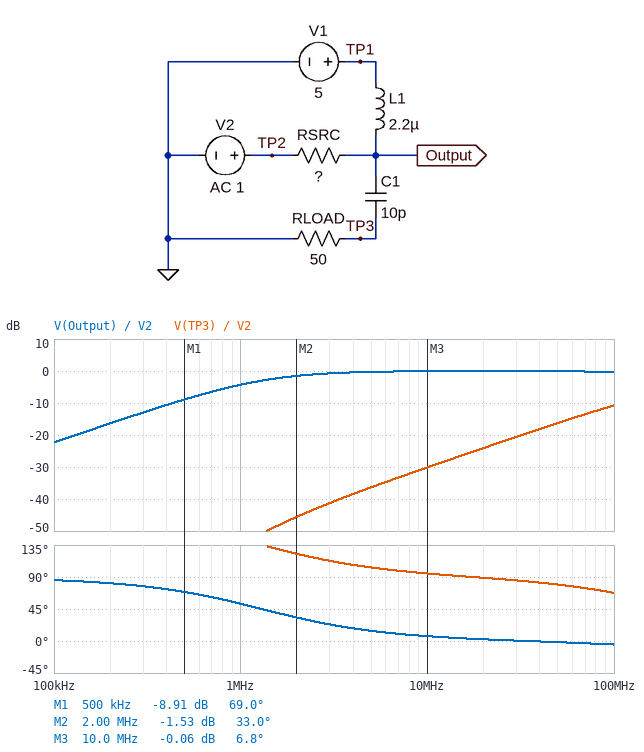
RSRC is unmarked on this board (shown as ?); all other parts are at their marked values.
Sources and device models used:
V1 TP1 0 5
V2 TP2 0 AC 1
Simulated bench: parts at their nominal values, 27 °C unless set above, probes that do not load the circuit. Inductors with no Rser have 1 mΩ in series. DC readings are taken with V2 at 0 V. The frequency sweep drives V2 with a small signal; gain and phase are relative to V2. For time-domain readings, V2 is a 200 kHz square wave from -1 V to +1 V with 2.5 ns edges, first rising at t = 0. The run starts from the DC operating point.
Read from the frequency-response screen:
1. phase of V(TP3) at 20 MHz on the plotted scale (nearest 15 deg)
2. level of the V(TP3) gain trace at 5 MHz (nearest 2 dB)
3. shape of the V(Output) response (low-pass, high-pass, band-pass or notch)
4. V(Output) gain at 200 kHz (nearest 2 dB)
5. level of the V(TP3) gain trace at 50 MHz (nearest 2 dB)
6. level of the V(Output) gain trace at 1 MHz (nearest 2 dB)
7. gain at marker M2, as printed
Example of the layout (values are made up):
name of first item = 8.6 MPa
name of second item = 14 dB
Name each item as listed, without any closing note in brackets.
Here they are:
phase of V(TP3) at 20 MHz on the plotted scale = 90 deg
level of the V(TP3) gain trace at 5 MHz = -36 dB
shape of the V(Output) response = high-pass
V(Output) gain at 200 kHz = -16 dB
level of the V(TP3) gain trace at 50 MHz = -16 dB
level of the V(Output) gain trace at 1 MHz = -4 dB
gain at marker M2, as printed = -1.53 dB
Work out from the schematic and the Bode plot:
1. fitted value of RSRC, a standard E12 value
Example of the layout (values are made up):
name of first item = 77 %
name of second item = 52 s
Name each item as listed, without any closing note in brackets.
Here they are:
fitted value of RSRC, a standard E12 value = 18 Ω
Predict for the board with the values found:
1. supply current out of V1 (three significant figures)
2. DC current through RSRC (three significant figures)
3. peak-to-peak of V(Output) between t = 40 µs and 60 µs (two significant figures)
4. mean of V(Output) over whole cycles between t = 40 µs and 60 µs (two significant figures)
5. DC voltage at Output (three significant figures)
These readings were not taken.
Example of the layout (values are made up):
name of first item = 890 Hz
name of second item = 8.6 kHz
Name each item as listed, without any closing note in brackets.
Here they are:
supply current out of V1 = 278 mA
DC current through RSRC = 278 mA
peak-to-peak of V(Output) between t = 40 µs and 60 µs = 3.9 V
mean of V(Output) over whole cycles between t = 40 µs and 60 µs = 5.0 V
DC voltage at Output = 5.00 V
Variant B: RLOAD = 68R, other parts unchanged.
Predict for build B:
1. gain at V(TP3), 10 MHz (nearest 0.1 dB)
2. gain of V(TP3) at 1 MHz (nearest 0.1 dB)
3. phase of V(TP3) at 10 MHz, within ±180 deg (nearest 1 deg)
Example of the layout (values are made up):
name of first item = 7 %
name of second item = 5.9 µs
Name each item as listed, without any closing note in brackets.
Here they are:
gain at V(TP3), 10 MHz = -27.5 dB
gain of V(TP3) at 1 MHz = -51.7 dB
phase of V(TP3) at 10 MHz, within ±180 deg = 94 deg
